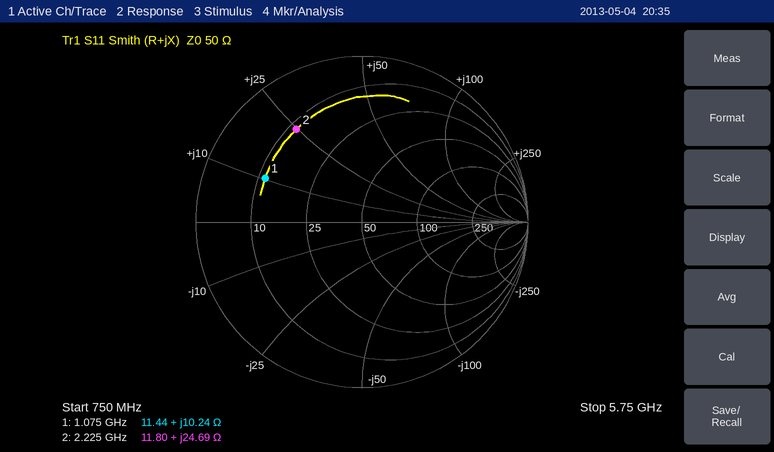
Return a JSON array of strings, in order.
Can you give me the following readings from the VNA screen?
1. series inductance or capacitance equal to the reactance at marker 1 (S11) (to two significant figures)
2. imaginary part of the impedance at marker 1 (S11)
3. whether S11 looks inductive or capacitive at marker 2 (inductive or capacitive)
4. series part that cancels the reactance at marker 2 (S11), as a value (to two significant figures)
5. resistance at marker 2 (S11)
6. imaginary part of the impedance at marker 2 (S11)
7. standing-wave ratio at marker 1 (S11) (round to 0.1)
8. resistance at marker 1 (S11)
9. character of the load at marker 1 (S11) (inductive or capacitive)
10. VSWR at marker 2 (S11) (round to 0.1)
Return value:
["1.5 nH", "+10.24 Ω", "inductive", "2.9 pF", "11.80 Ω", "+24.69 Ω", "4.6", "11.44 Ω", "inductive", "5.3"]
